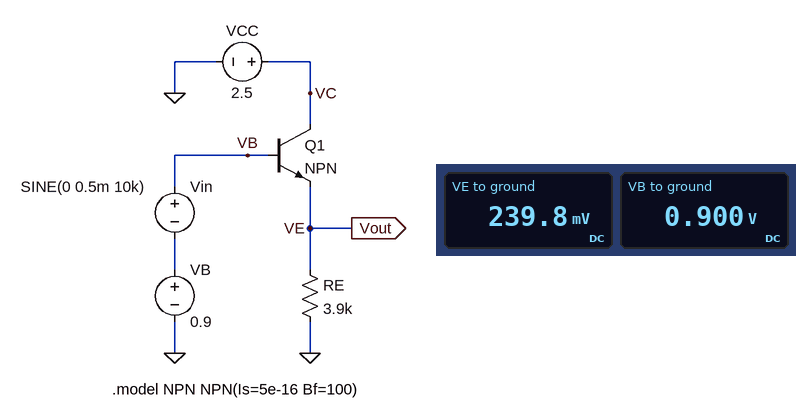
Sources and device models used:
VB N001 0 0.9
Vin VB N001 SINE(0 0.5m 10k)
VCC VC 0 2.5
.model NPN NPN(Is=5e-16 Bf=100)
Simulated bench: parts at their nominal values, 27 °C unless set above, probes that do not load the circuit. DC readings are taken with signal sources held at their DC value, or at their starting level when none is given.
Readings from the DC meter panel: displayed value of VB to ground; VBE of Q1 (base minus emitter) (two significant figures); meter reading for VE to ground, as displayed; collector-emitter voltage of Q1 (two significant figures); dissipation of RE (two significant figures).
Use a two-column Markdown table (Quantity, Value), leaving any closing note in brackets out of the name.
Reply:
| Quantity | Value |
|---|---|
| displayed value of VB to ground | 0.900 V |
| VBE of Q1 (base minus emitter) | 660 mV |
| meter reading for VE to ground, as displayed | 239.8 mV |
| collector-emitter voltage of Q1 | 2.3 V |
| dissipation of RE | 15 µW |
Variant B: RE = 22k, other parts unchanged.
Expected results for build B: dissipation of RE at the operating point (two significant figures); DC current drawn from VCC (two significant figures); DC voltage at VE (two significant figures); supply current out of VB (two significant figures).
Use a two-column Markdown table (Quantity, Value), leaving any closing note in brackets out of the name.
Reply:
| Quantity | Value |
|---|---|
| dissipation of RE at the operating point | 3.6 µW |
| DC current drawn from VCC | 13 µA |
| DC voltage at VE | 280 mV |
| supply current out of VB | 130 nA |
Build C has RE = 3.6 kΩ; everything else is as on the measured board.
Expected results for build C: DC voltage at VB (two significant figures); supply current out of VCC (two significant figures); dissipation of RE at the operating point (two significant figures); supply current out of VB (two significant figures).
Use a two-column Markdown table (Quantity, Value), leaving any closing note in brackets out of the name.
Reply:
| Quantity | Value |
|---|---|
| DC voltage at VB | 900 mV |
| supply current out of VCC | 65 µA |
| dissipation of RE at the operating point | 16 µW |
| supply current out of VB | 650 nA |
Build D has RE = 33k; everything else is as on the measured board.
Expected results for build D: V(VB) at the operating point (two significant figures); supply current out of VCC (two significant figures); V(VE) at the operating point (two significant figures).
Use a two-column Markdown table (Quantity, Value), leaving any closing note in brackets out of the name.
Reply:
| Quantity | Value |
|---|---|
| V(VB) at the operating point | 900 mV |
| supply current out of VCC | 8.7 µA |
| V(VE) at the operating point | 290 mV |
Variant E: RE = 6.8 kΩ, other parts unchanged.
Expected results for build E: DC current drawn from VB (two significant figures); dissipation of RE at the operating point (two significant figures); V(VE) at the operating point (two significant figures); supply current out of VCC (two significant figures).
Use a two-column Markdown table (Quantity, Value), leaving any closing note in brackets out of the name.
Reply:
| Quantity | Value |
|---|---|
| DC current drawn from VB | 370 nA |
| dissipation of RE at the operating point | 9.4 µW |
| V(VE) at the operating point | 250 mV |
| supply current out of VCC | 37 µA |
